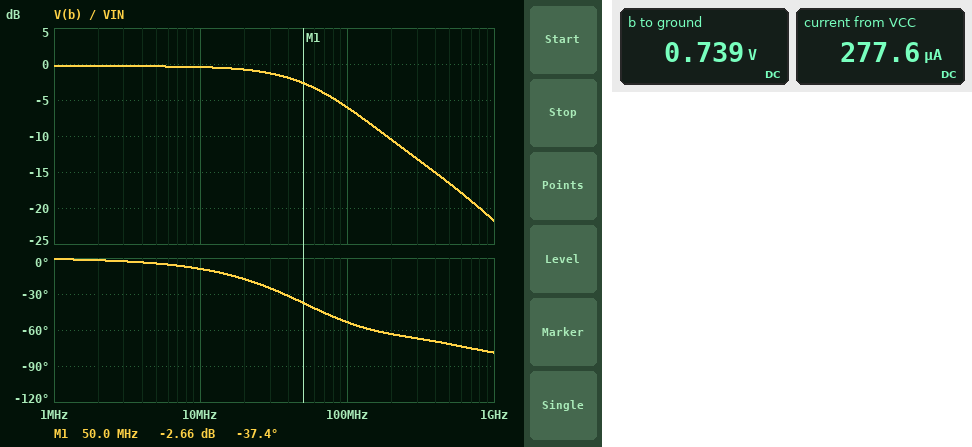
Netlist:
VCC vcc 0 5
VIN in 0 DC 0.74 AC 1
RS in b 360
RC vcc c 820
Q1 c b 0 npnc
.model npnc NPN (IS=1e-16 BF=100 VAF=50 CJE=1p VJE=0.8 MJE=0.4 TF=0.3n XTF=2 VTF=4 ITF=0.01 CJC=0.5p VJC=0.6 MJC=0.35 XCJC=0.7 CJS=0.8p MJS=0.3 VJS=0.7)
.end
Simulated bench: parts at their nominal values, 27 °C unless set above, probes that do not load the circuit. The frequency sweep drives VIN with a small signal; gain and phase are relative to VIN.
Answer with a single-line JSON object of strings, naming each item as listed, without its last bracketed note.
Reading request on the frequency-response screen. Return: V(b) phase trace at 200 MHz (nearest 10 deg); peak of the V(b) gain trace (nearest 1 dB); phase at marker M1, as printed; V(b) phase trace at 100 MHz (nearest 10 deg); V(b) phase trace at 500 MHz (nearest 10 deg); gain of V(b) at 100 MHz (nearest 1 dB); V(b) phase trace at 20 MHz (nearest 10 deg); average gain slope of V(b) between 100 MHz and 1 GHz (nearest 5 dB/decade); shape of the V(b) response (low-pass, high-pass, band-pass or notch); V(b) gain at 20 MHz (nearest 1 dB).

{"V(b) phase trace at 200 MHz": "-60 deg", "peak of the V(b) gain trace": "0 dB", "phase at marker M1, as printed": "-37.4 deg", "V(b) phase trace at 100 MHz": "-50 deg", "V(b) phase trace at 500 MHz": "-70 deg", "gain of V(b) at 100 MHz": "-6 dB", "V(b) phase trace at 20 MHz": "-20 deg", "average gain slope of V(b) between 100 MHz and 1 GHz": "-15 dB/decade", "shape of the V(b) response": "low-pass", "V(b) gain at 20 MHz": "-1 dB"}
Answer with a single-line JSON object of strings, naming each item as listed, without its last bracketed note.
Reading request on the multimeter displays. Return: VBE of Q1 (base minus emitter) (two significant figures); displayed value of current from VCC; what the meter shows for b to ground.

{"VBE of Q1 (base minus emitter)": "740 mV", "displayed value of current from VCC": "277.6 µA", "what the meter shows for b to ground": "0.739 V"}
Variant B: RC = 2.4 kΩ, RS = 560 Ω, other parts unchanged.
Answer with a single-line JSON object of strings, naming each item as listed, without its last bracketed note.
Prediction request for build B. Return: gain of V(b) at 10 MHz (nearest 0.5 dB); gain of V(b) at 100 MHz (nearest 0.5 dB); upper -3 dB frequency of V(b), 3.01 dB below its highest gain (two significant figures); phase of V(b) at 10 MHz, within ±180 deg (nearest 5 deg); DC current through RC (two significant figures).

{"gain of V(b) at 10 MHz": "-1.0 dB", "gain of V(b) at 100 MHz": "-11.0 dB", "upper -3 dB frequency of V(b), 3.01 dB below its highest gain": "24 MHz", "phase of V(b) at 10 MHz, within ±180 deg": "-20 deg", "DC current through RC": "270 µA"}
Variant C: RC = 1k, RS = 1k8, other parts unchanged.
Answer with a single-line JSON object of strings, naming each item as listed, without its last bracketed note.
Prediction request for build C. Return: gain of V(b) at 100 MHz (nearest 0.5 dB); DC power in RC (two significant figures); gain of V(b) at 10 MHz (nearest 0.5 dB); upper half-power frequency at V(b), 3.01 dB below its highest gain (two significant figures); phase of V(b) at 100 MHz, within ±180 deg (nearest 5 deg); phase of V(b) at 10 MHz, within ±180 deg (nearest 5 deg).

{"gain of V(b) at 100 MHz": "-18.0 dB", "DC power in RC": "60 µW", "gain of V(b) at 10 MHz": "-3.0 dB", "upper half-power frequency at V(b), 3.01 dB below its highest gain": "14 MHz", "phase of V(b) at 100 MHz, within ±180 deg": "-75 deg", "phase of V(b) at 10 MHz, within ±180 deg": "-35 deg"}
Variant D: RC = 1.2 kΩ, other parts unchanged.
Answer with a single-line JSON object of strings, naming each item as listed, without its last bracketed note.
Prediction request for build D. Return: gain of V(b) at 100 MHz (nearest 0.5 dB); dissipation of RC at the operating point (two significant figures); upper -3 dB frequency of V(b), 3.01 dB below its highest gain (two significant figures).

{"gain of V(b) at 100 MHz": "-7.0 dB", "dissipation of RC at the operating point": "92 µW", "upper -3 dB frequency of V(b), 3.01 dB below its highest gain": "51 MHz"}
